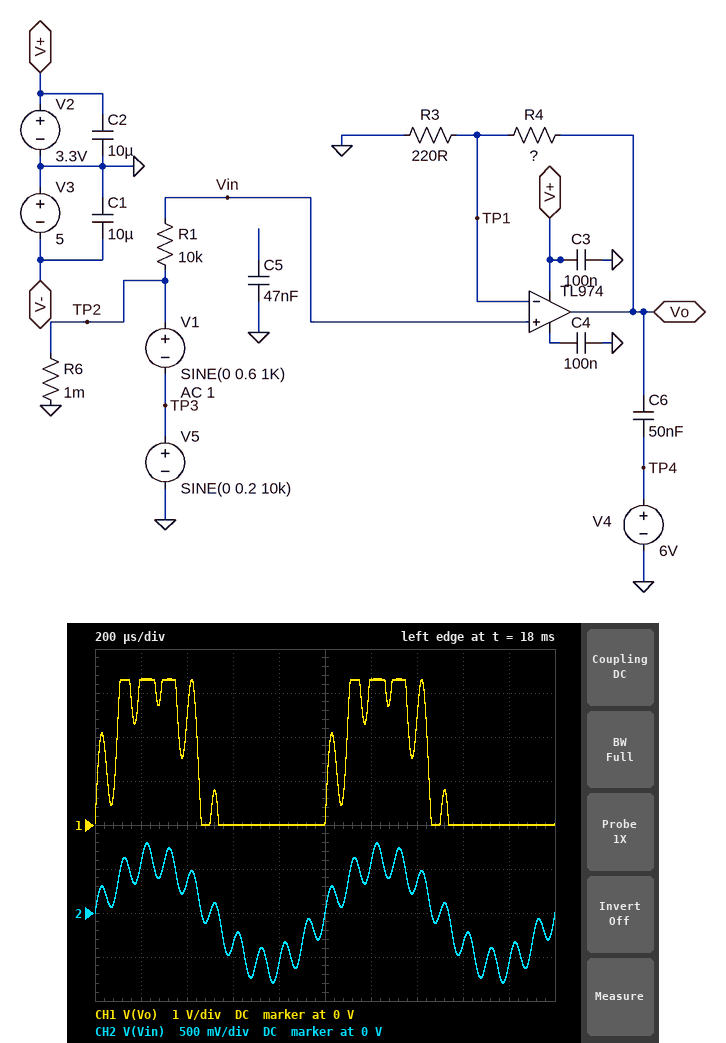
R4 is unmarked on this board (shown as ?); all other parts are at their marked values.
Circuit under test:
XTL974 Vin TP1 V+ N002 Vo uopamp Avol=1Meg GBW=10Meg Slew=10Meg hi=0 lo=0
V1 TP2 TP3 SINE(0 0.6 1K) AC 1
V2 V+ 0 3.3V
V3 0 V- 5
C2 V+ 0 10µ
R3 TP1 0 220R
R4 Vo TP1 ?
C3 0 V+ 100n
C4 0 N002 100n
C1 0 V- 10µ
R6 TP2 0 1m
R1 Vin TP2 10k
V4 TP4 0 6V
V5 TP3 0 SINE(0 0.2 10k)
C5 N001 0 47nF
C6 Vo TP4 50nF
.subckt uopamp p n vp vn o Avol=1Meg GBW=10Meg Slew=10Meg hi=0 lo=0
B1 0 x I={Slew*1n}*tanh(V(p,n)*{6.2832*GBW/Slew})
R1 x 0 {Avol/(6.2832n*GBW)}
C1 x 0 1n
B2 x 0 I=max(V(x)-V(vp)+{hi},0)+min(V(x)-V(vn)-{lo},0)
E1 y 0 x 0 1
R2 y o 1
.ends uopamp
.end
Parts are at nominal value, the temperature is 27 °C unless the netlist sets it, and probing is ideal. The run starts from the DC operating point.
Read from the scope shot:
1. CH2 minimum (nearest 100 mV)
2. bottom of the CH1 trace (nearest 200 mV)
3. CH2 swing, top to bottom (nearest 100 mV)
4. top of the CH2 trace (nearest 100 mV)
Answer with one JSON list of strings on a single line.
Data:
["-800 mV", "0 V", "1.6 V", "800 mV"]
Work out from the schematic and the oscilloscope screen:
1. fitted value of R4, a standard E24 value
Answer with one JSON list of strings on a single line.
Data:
["1.3 kΩ"]
